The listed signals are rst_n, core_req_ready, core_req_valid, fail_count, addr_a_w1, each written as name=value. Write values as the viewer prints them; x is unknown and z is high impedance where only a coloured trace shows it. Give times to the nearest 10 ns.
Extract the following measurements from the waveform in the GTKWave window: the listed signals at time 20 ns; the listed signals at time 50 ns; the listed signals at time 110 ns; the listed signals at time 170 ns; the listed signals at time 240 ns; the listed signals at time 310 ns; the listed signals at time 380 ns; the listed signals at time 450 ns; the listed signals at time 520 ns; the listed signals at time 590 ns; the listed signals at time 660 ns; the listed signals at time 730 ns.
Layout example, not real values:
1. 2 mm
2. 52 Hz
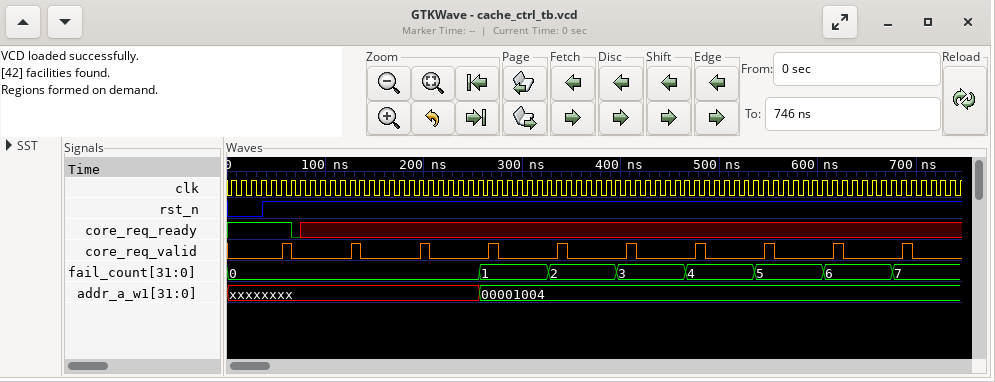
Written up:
1. rst_n=0, core_req_ready=1, core_req_valid=0, fail_count=0, addr_a_w1=xxxxxxxx
2. rst_n=1, core_req_ready=1, core_req_valid=0, fail_count=0, addr_a_w1=xxxxxxxx
3. rst_n=1, core_req_ready=x, core_req_valid=0, fail_count=0, addr_a_w1=xxxxxxxx
4. rst_n=1, core_req_ready=x, core_req_valid=0, fail_count=0, addr_a_w1=xxxxxxxx
5. rst_n=1, core_req_ready=x, core_req_valid=0, fail_count=0, addr_a_w1=xxxxxxxx
6. rst_n=1, core_req_ready=x, core_req_valid=0, fail_count=1, addr_a_w1=00001004
7. rst_n=1, core_req_ready=x, core_req_valid=0, fail_count=2, addr_a_w1=00001004
8. rst_n=1, core_req_ready=x, core_req_valid=0, fail_count=3, addr_a_w1=00001004
9. rst_n=1, core_req_ready=x, core_req_valid=0, fail_count=4, addr_a_w1=00001004
10. rst_n=1, core_req_ready=x, core_req_valid=0, fail_count=5, addr_a_w1=00001004
11. rst_n=1, core_req_ready=x, core_req_valid=0, fail_count=6, addr_a_w1=00001004
12. rst_n=1, core_req_ready=x, core_req_valid=0, fail_count=7, addr_a_w1=00001004
